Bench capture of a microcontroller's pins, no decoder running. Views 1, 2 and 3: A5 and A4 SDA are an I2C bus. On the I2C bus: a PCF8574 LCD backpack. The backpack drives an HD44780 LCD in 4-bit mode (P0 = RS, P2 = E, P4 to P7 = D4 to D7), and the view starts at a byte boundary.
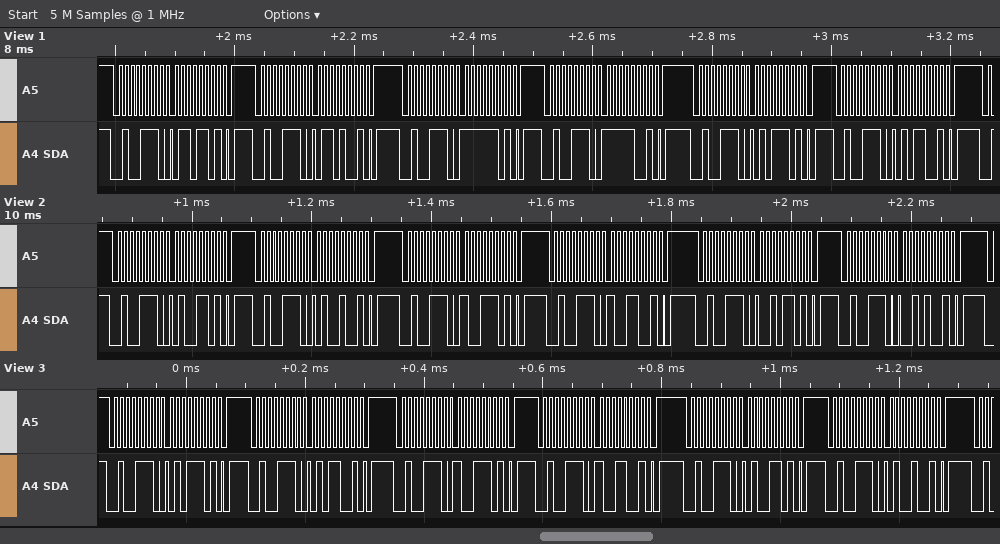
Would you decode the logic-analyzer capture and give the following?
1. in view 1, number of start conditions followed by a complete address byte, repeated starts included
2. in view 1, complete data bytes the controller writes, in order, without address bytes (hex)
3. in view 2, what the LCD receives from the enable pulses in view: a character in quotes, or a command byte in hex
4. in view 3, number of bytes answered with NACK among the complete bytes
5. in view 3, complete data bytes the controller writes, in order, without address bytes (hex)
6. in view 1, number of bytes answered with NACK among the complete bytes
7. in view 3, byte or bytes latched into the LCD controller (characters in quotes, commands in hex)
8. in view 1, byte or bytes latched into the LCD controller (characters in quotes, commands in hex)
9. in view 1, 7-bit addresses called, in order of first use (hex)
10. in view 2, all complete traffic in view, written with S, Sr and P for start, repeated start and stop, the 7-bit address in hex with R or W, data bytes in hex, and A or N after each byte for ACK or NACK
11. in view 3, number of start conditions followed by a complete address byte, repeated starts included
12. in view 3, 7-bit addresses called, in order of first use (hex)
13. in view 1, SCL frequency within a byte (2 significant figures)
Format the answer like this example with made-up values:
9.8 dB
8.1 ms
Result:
6
6D 69 FD F9 5D 59
'I'
0
5D 59 9D 99 4D 49
0
'Y'
'o'
0x27
S 27W A 4D A P S 27W A 49 A P S 27W A 9D A P S 27W A 99 A P S 27W A 2D A P S 27W A 29 A P
6
0x27
100 kHz
